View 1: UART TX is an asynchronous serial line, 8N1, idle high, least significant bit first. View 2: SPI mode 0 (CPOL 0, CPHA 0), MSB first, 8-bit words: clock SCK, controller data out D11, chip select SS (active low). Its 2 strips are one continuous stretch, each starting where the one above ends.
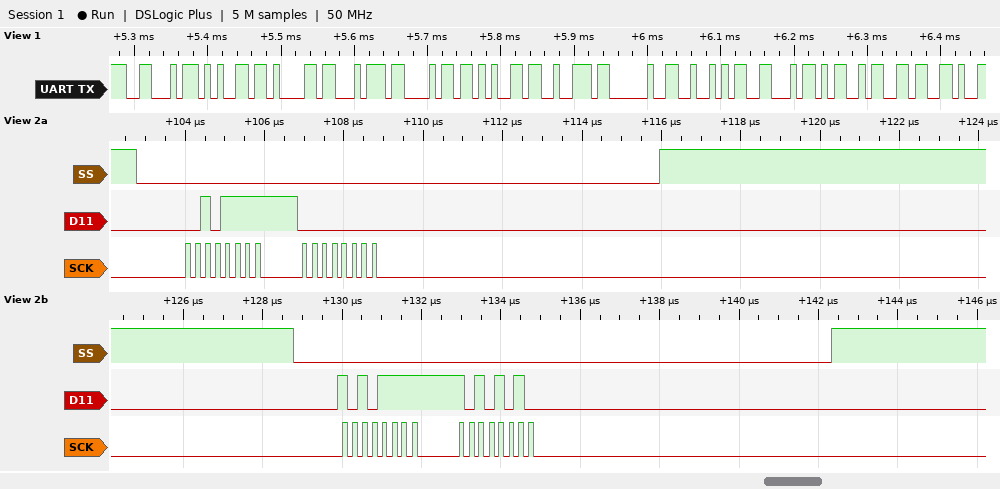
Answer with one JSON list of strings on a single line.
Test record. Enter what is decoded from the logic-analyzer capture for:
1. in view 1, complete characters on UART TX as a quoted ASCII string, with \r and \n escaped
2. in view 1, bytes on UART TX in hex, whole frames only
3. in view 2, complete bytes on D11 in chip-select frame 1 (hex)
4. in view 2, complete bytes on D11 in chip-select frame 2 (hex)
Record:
["\"Feather RFM6\"", "0x46 0x65 0x61 0x74 0x68 0x65 0x72 0x20 0x52 0x46 0x4D 0x36", "2F 00", "AF AA"]
